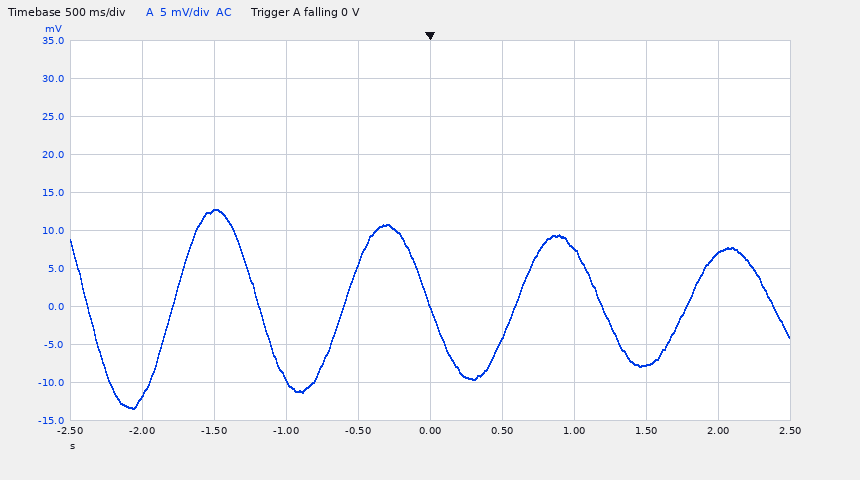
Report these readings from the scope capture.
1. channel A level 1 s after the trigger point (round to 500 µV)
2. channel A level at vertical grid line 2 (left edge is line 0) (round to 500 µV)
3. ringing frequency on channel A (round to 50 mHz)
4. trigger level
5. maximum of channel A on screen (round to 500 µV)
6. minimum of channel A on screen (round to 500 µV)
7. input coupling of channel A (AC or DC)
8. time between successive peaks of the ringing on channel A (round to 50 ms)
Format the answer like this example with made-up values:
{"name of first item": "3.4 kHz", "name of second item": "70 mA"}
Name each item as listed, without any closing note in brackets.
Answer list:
{"channel A level 1 s after the trigger point": "7.5 mV", "channel A level at vertical grid line 2 (left edge is line 0)": "12.5 mV", "ringing frequency on channel A": "850 mHz", "trigger level": "0 V", "maximum of channel A on screen": "13.0 mV", "minimum of channel A on screen": "-13.5 mV", "input coupling of channel A": "AC", "time between successive peaks of the ringing on channel A": "1.20 s"}
